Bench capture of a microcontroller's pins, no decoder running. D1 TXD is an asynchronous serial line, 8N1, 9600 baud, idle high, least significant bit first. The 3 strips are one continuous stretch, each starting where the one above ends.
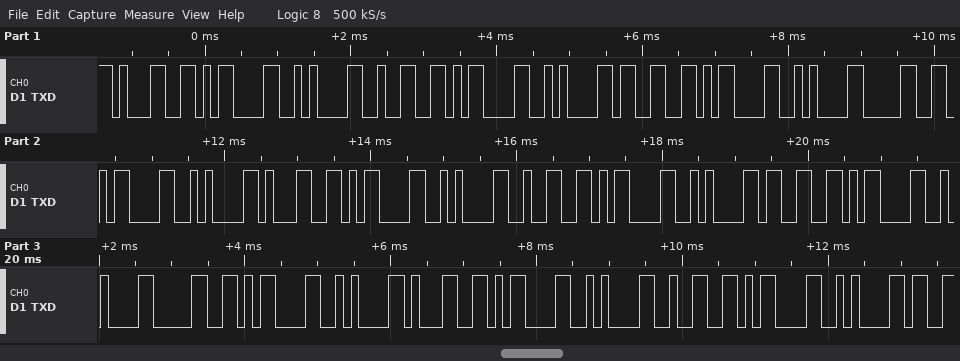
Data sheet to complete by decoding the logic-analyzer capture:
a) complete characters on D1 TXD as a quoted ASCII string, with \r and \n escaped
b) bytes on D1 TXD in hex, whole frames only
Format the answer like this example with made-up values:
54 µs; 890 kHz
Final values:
"1\r\n2\r\n3\r\n0\r\n1\r\n2\r\n3\r\n0\r\n1\r\n2\r\n"; 31 0D 0A 32 0D 0A 33 0D 0A 30 0D 0A 31 0D 0A 32 0D 0A 33 0D 0A 30 0D 0A 31 0D 0A 32 0D 0A
